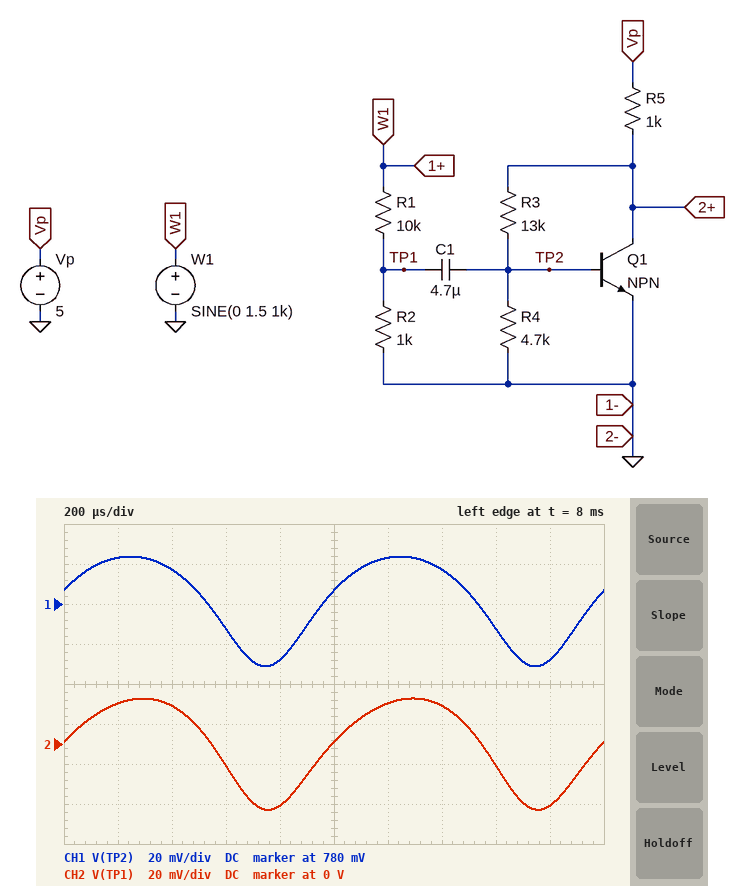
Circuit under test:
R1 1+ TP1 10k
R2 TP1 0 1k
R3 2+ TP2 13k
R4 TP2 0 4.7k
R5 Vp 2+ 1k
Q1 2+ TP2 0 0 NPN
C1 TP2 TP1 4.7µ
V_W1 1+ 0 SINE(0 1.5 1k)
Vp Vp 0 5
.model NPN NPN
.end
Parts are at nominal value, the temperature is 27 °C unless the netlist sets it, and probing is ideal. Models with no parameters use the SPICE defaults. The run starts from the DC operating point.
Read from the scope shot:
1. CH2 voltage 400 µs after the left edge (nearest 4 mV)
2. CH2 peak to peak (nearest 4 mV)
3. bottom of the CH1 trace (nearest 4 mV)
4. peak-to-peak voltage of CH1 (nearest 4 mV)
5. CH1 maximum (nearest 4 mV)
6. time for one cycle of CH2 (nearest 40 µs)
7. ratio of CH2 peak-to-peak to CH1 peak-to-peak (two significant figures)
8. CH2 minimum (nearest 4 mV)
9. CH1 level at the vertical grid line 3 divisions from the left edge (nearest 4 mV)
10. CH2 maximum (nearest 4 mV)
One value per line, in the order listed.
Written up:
20 mV
56 mV
748 mV
56 mV
804 mV
1.00 ms
1.0
-32 mV
768 mV
24 mV
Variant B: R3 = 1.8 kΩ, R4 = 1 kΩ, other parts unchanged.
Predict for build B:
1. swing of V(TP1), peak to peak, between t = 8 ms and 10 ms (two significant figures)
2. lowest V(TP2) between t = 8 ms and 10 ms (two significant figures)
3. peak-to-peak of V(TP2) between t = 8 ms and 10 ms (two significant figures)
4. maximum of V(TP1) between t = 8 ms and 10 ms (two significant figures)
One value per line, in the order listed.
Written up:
14 mV
790 mV
10 mV
7.7 mV
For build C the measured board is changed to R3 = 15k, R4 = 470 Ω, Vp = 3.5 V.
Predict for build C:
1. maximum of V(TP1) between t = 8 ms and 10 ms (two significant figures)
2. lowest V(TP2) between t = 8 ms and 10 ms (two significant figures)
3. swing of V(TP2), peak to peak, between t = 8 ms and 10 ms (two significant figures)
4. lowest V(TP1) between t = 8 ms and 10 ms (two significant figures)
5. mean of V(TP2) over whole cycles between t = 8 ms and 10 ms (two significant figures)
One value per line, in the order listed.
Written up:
46 mV
54 mV
91 mV
-45 mV
100 mV
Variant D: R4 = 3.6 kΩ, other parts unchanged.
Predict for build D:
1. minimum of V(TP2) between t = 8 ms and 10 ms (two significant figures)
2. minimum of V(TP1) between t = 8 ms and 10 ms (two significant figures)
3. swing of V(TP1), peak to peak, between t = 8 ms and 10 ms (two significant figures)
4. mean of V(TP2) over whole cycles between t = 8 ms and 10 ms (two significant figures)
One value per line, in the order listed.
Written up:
720 mV
-48 mV
79 mV
770 mV
